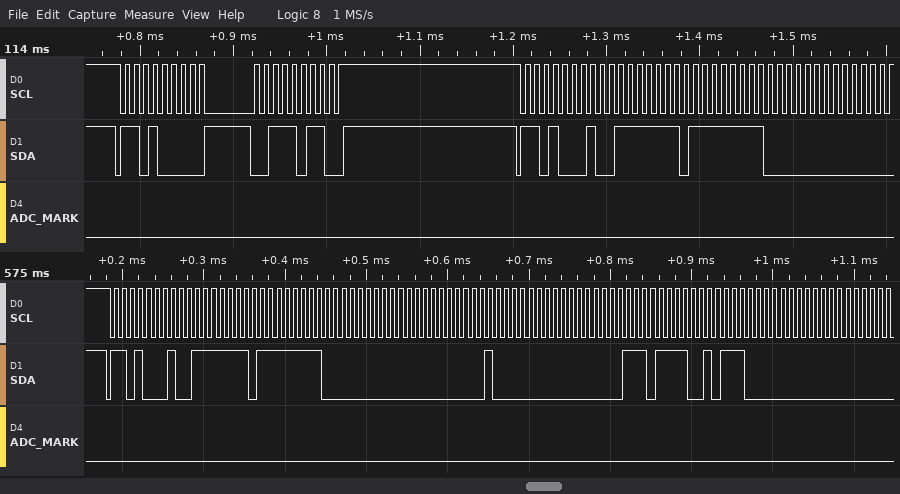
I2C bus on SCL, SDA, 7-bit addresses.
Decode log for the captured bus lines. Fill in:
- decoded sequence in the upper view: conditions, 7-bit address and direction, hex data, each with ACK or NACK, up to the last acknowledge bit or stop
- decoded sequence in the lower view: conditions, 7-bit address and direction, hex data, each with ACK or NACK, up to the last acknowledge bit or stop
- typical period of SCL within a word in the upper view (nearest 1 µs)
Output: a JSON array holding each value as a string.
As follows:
["start, address 68 write ACK, 3B ACK, stop, start, address 68 read ACK, 7F ACK, FF ACK, 00 ACK", "start, address 68 read ACK, 7F ACK, FF ACK, 00 ACK, 00 ACK, 40 ACK, 00 ACK, EF ACK, 5C ACK, 00 ACK", "10 µs"]
